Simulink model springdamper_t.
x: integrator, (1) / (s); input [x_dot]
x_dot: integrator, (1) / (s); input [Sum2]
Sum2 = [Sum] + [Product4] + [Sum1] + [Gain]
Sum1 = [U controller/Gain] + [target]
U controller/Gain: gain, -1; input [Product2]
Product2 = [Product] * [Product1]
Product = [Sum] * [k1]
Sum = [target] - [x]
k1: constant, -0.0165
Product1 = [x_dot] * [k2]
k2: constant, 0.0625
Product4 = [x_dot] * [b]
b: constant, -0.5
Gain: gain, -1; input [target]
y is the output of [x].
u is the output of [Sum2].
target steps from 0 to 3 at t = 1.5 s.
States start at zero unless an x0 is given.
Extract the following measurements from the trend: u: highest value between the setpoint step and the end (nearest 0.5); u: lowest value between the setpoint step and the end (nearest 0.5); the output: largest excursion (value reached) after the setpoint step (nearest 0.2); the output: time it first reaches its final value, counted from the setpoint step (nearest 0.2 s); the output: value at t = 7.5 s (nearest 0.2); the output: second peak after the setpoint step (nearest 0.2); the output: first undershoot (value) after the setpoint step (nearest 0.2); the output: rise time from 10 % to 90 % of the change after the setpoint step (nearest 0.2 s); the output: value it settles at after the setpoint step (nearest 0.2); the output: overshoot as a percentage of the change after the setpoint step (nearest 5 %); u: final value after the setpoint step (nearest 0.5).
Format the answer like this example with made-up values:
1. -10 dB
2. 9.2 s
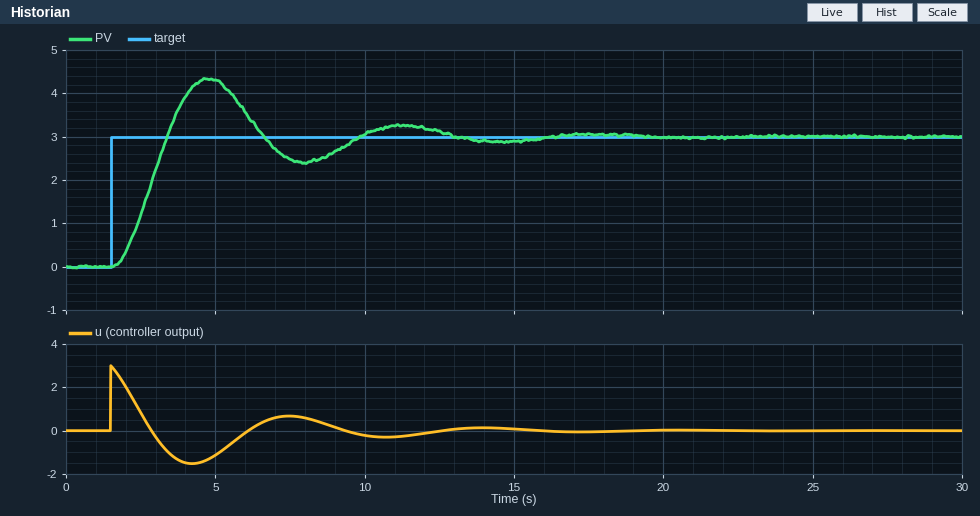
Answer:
1. 3.0
2. -1.5
3. 4.4
4. 1.8 s
5. 2.4
6. 3.2
7. 2.4
8. 1.2 s
9. 3.0
10. 45 %
11. 0.0
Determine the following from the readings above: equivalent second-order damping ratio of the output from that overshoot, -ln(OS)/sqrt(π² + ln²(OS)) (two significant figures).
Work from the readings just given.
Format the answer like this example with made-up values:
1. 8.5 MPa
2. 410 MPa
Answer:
1. 0.25
